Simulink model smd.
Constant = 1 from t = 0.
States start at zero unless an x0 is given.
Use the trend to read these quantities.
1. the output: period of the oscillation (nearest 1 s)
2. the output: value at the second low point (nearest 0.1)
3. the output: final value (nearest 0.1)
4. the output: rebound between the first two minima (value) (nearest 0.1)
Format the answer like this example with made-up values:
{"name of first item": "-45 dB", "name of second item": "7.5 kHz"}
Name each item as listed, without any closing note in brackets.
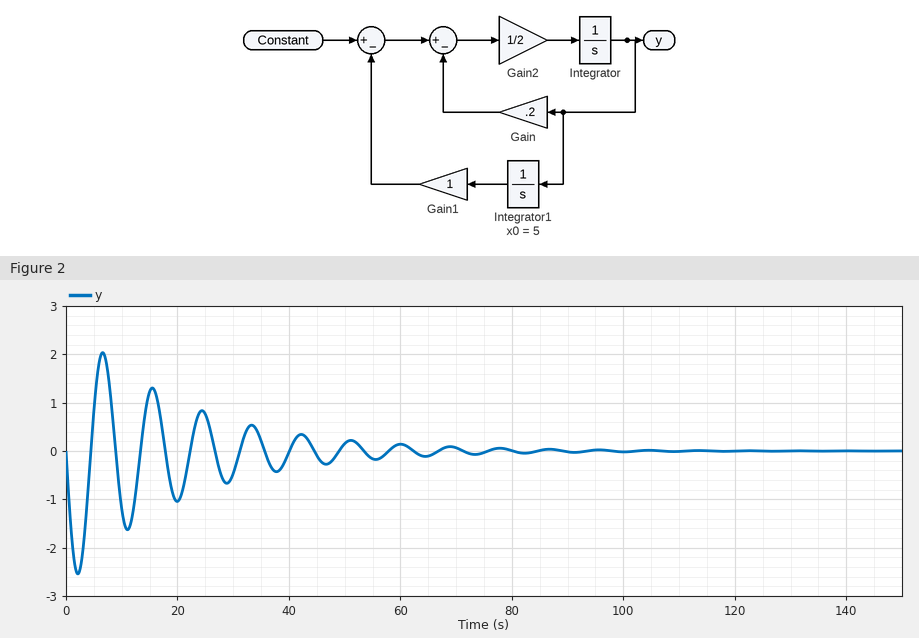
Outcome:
{"the output: period of the oscillation": "9 s", "the output: value at the second low point": "-1.6", "the output: final value": "0.0", "the output: rebound between the first two minima (value)": "2.0"}
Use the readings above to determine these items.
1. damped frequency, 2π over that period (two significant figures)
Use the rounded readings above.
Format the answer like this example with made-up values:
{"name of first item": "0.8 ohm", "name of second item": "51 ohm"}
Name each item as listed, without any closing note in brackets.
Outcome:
{"damped frequency, 2π over that period": "0.70 rad/s"}
